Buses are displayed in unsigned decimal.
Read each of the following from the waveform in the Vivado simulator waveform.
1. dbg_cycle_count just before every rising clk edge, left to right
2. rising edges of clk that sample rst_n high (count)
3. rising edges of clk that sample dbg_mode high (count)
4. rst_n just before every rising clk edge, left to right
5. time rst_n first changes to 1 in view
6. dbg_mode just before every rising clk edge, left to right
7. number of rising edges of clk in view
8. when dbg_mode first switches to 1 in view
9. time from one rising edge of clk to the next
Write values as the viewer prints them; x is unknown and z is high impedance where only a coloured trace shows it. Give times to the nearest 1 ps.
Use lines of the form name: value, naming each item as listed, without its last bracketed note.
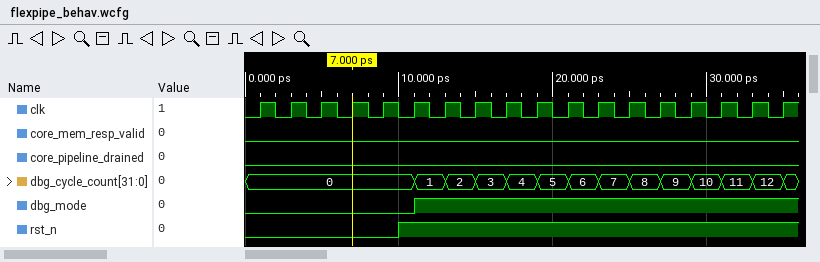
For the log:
dbg_cycle_count just before every rising clk edge, left to right: 0, 0, 0, 0, 0, 0, 1, 2, 3, 4, 5, 6, 7, 8, 9, 10, 11, 12
rising edges of clk that sample rst_n high: 13
rising edges of clk that sample dbg_mode high: 12
rst_n just before every rising clk edge, left to right: 0 0 0 0 0 1 1 1 1 1 1 1 1 1 1 1 1 1
time rst_n first changes to 1 in view: 10 ps
dbg_mode just before every rising clk edge, left to right: 0 0 0 0 0 0 1 1 1 1 1 1 1 1 1 1 1 1
number of rising edges of clk in view: 18
when dbg_mode first switches to 1 in view: 11 ps
time from one rising edge of clk to the next: 2 ps
